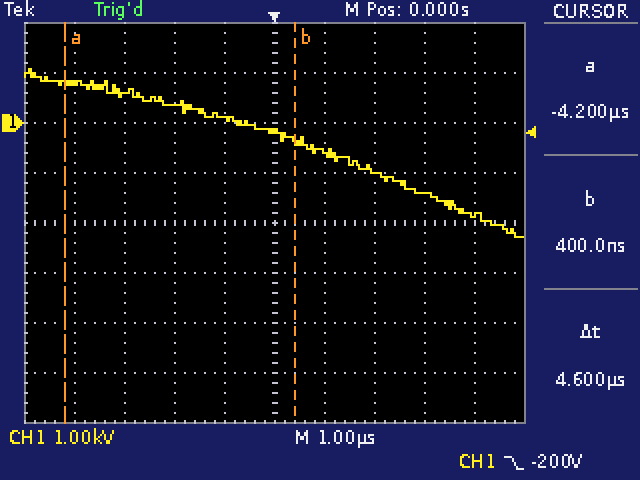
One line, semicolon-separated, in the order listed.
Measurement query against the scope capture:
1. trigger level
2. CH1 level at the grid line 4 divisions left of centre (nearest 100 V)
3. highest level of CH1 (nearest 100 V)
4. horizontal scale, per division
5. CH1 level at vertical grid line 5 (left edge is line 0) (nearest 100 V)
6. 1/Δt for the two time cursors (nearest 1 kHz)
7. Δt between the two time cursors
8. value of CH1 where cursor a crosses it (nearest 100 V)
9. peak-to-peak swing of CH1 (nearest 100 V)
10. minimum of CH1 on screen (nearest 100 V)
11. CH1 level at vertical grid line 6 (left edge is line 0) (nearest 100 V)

-200 V; 800 V; 1.1 kV; 1 µs; -200 V; 217 kHz; 4.6 µs; 800 V; 3.4 kV; -2.3 kV; -600 V
